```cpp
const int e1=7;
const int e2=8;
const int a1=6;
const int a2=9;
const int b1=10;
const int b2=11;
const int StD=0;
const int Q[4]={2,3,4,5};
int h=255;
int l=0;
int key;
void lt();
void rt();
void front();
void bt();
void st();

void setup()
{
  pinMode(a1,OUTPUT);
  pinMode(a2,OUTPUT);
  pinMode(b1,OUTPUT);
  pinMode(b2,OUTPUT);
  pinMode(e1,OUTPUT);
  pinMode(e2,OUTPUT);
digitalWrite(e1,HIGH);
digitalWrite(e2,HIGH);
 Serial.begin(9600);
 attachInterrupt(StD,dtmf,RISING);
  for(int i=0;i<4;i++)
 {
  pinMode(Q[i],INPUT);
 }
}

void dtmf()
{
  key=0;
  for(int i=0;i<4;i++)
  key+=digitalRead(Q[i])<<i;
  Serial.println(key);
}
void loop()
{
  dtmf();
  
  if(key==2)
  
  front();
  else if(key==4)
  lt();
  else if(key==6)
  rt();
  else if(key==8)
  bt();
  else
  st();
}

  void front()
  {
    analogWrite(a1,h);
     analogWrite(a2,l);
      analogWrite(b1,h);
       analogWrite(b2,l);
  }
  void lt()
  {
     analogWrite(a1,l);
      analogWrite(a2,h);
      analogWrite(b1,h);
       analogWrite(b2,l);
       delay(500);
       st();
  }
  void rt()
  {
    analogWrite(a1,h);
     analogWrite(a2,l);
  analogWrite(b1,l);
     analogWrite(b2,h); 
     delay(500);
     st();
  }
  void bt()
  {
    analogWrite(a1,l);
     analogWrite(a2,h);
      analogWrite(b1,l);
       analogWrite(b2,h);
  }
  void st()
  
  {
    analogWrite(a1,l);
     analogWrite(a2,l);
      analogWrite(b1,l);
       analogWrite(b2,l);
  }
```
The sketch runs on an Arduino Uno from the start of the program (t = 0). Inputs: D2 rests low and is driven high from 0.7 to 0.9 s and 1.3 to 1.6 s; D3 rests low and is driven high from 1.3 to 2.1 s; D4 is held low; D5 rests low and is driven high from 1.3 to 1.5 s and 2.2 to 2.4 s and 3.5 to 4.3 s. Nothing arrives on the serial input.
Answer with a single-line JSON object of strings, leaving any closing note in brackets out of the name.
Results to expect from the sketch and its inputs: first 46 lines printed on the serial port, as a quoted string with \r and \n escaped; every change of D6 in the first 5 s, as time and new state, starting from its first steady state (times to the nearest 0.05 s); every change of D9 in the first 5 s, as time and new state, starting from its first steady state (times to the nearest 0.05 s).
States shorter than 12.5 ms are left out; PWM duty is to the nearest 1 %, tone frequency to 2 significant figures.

{"first 46 lines printed on the serial port, as a quoted string with \\r and \\n escaped": "\"0\\r\\n0\\r\\n0\\r\\n0\\r\\n0\\r\\n0\\r\\n0\\r\\n0\\r\\n0\\r\\n0\\r\\n0\\r\\n0\\r\\n0\\r\\n0\\r\\n0\\r\\n0\\r\\n0\\r\\n0\\r\\n0\\r\\n0\\r\\n0\\r\\n0\\r\\n0\\r\\n0\\r\\n0\\r\\n0\\r\\n0\\r\\n0\\r\\n0\\r\\n0\\r\\n0\\r\\n0\\r\\n0\\r\\n0\\r\\n0\\r\\n0\\r\\n0\\r\\n0\\r\\n0\\r\\n0\\r\\n0\\r\\n0\\r\\n0\\r\\n0\\r\\n0\\r\\n0\\r\\n\"", "every change of D6 in the first 5 s, as time and new state, starting from its first steady state": "0 s low; 1.6 s high; 2.1 s low", "every change of D9 in the first 5 s, as time and new state, starting from its first steady state": "0 s low; 2.2 s high; 2.4 s low; 3.5 s high; 4.3 s low"}
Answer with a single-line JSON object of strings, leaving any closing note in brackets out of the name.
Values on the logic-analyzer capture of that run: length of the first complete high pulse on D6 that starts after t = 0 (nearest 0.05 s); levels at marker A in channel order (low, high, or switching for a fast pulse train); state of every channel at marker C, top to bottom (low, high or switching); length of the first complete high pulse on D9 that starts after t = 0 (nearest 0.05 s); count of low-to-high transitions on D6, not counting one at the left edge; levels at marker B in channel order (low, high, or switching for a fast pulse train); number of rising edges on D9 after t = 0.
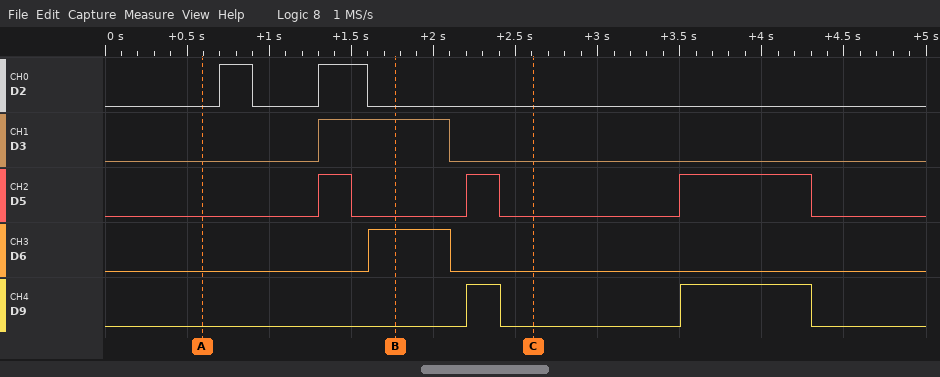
{"length of the first complete high pulse on D6 that starts after t = 0": "0.50 s", "levels at marker A in channel order": "D2 low, D3 low, D5 low, D6 low, D9 low", "state of every channel at marker C, top to bottom": "D2 low, D3 low, D5 low, D6 low, D9 low", "length of the first complete high pulse on D9 that starts after t = 0": "0.20 s", "count of low-to-high transitions on D6, not counting one at the left edge": "1", "levels at marker B in channel order": "D2 low, D3 high, D5 low, D6 high, D9 low", "number of rising edges on D9 after t = 0": "2"}
